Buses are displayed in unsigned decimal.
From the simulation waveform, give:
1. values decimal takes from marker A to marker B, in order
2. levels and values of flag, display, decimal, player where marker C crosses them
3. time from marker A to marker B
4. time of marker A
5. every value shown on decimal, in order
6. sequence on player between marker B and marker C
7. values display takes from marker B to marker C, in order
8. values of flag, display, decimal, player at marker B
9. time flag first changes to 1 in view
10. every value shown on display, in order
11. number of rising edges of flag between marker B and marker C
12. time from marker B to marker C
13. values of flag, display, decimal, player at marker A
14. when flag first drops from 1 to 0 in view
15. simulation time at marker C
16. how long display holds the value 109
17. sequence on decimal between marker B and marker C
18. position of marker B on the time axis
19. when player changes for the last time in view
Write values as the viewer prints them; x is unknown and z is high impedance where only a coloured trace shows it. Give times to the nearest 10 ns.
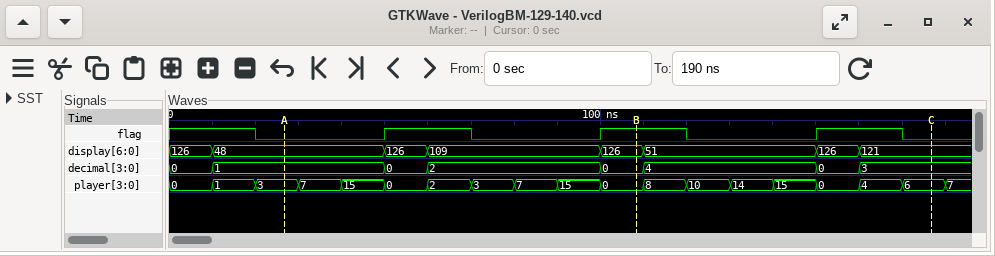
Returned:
1, 0, 2, 0
flag=0, display=121, decimal=3, player=6
80 ns
30 ns
0, 1, 0, 2, 0, 4, 0, 3
0, 8, 10, 14, 15, 0, 4, 6
126, 51, 126, 121
flag=1, display=126, decimal=0, player=0
50 ns
126, 48, 126, 109, 126, 51, 126, 121
1
70 ns
flag=0, display=48, decimal=1, player=3
20 ns
180 ns
40 ns
0, 4, 0, 3
110 ns
180 ns
